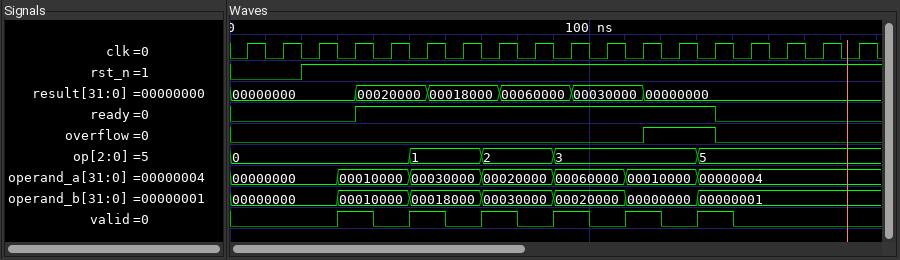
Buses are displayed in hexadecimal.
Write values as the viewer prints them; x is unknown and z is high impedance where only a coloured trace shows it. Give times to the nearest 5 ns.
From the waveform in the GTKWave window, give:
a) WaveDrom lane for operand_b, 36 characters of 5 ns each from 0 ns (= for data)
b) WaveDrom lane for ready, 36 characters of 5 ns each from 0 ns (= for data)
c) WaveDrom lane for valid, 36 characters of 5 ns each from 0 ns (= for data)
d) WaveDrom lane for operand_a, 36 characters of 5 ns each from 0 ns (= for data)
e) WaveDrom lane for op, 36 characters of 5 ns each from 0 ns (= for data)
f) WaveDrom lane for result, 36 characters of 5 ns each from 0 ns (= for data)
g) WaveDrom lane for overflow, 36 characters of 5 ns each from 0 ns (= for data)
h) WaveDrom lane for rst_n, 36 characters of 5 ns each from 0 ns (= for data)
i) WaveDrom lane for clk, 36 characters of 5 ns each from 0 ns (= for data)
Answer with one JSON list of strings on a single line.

["{name: 'operand_b', wave: '=.....=...=...=...=...=...=.........', data: '00000000 00010000 00018000 00030000 00020000 00000000 00000001'}", "{name: 'ready', wave: '0......1...................0........'}", "{name: 'valid', wave: '0.....1.0.1.0.1.0.1.0.1.0.1.0.......'}", "{name: 'operand_a', wave: '=.....=...=...=...=...=...=.........', data: '00000000 00010000 00030000 00020000 00060000 00010000 00000004'}", "{name: 'op', wave: '=.........=...=...=.......=.........', data: '0 1 2 3 5'}", "{name: 'result', wave: '=......=...=...=...=...=............', data: '00000000 00020000 00018000 00060000 00030000 00000000'}", "{name: 'overflow', wave: '0......................1...0........'}", "{name: 'rst_n', wave: '0...1...............................'}", "{name: 'clk', wave: '010101010101010101010101010101010101'}"]
